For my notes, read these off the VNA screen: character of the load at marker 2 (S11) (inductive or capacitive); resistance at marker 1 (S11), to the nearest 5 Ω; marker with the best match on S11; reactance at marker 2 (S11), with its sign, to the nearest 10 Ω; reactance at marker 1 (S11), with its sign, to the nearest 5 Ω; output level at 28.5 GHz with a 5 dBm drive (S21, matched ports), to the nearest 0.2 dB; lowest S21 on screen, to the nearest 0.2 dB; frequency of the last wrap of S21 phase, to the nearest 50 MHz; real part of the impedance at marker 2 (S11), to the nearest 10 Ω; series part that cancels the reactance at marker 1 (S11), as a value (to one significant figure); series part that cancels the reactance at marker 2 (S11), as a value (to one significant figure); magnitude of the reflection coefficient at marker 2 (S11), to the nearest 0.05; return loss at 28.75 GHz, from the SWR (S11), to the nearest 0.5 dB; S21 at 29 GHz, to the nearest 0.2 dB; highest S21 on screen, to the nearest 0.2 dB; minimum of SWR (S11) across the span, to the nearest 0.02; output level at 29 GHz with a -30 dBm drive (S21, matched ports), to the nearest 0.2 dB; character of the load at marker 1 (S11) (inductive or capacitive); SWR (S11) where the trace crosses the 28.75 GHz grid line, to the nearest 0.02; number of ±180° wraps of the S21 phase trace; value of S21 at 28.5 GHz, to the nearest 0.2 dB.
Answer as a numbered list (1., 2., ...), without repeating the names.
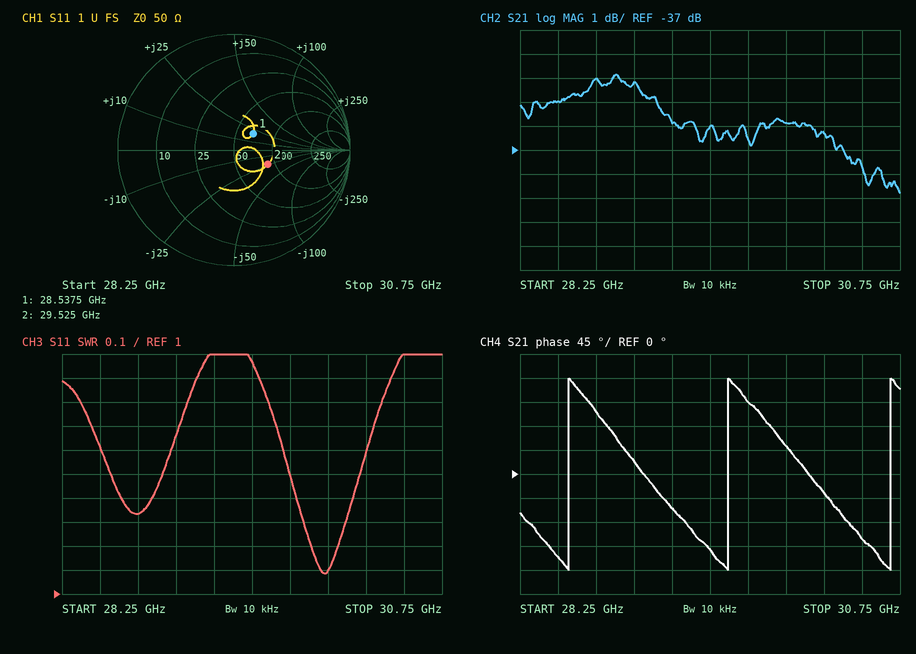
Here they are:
1. capacitive
2. 65 Ω
3. marker 1
4. -20 Ω
5. +20 Ω
6. -30.0 dBm
7. -38.8 dB
8. 30.70 GHz
9. 90 Ω
10. 300 fF
11. 100 pH
12. 0.30
13. 17.0 dB
14. -34.2 dB
15. -33.8 dB
16. 1.08
17. -64.2 dBm
18. inductive
19. 1.34
20. 3
21. -35.0 dB
